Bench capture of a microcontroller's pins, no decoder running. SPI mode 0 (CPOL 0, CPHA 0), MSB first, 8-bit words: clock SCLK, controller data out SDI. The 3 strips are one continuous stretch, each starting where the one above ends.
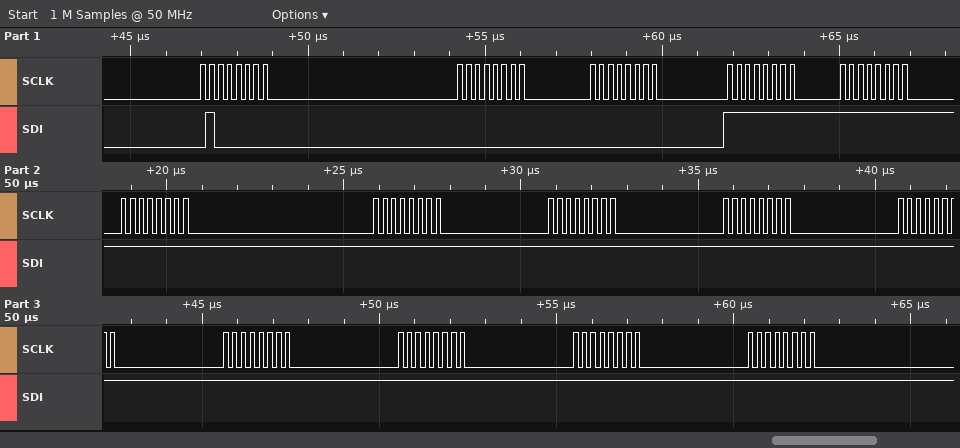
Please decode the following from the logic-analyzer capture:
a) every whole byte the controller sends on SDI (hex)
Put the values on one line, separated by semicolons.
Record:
40 00 00 FF FF FF FF FF FF FF FF FF FF FF
